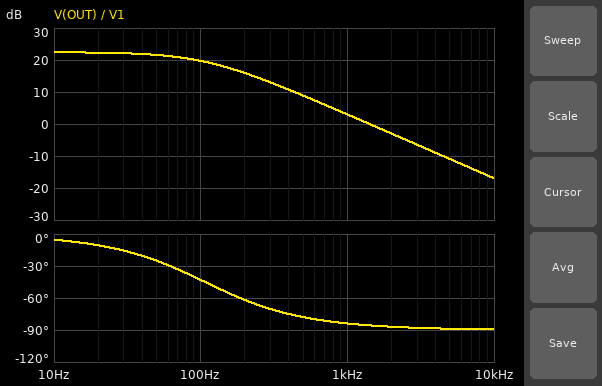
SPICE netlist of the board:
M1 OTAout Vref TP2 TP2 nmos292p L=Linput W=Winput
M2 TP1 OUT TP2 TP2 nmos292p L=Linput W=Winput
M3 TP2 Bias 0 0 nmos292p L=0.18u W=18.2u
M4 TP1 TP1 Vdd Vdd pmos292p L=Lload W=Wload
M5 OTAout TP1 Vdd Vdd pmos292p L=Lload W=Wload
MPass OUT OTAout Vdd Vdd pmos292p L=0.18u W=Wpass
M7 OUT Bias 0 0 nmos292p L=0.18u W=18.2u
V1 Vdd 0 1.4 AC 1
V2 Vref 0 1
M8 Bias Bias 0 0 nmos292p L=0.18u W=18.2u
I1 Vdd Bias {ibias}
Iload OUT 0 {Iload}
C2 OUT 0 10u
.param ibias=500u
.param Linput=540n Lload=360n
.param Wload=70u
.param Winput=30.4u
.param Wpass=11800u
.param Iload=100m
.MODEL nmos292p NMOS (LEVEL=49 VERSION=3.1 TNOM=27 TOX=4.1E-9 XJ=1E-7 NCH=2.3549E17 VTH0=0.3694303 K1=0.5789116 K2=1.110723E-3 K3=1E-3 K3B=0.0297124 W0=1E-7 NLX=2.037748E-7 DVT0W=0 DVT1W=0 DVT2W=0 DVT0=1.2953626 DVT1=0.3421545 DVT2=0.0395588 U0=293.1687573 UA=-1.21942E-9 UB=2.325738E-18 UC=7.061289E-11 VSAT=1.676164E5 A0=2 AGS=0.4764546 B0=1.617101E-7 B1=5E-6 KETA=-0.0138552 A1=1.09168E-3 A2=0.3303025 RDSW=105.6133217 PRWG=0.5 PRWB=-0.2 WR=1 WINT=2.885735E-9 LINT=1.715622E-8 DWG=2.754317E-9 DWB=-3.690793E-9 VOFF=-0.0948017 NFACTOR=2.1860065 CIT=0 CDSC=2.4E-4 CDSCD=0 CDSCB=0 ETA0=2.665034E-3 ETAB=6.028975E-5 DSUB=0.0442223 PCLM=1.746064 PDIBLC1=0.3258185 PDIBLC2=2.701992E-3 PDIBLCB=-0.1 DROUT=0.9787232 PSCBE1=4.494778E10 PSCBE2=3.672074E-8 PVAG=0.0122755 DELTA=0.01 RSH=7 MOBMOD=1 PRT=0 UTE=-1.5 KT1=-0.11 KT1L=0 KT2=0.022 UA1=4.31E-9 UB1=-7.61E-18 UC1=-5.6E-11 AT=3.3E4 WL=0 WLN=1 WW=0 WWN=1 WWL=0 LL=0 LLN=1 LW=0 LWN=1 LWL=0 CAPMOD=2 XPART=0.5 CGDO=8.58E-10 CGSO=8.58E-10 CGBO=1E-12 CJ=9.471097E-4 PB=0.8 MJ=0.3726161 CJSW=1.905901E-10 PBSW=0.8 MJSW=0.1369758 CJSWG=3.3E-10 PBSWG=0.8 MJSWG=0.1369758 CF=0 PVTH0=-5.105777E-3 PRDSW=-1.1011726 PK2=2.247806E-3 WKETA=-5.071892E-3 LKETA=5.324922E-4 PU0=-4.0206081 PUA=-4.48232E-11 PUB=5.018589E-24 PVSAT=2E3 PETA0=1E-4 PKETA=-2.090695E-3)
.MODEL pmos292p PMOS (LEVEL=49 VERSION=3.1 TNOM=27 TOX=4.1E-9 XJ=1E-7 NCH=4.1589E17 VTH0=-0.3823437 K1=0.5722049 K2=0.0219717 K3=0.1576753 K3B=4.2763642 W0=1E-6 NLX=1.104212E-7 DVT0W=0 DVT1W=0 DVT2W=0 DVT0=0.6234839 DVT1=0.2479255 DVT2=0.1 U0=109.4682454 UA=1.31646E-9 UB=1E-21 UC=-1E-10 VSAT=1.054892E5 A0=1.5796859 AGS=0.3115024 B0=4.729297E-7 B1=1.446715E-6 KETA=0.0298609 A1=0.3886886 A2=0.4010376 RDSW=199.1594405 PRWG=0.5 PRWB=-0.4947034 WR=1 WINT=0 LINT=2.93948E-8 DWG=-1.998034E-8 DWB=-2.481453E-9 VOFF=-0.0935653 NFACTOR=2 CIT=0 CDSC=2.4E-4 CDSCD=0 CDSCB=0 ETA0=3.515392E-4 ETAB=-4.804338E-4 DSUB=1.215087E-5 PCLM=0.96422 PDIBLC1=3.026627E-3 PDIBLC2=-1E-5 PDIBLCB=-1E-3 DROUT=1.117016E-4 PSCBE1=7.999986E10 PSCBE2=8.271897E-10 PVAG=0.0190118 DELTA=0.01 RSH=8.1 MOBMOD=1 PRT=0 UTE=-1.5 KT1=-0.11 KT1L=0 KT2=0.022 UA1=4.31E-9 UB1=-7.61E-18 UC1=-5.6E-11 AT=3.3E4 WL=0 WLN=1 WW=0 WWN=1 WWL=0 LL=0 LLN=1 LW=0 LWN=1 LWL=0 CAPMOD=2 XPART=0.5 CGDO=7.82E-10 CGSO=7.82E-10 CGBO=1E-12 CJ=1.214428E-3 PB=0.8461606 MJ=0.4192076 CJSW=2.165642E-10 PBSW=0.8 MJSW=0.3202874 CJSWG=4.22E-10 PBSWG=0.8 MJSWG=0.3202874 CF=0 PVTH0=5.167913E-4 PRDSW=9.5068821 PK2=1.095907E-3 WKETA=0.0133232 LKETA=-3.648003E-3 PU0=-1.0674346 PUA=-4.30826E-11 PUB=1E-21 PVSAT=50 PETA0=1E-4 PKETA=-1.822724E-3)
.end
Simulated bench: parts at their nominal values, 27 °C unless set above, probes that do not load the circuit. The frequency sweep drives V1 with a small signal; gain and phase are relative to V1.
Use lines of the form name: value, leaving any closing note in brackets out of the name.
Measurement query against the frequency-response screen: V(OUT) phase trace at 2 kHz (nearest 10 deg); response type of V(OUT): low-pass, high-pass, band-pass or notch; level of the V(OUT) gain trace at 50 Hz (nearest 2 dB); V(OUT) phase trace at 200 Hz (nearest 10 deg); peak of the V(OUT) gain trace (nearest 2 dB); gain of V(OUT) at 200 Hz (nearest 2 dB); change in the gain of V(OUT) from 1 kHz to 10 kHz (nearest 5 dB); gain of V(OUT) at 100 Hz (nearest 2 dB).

V(OUT) phase trace at 2 kHz: -90 deg
response type of V(OUT): low-pass, high-pass, band-pass or notch: low-pass
level of the V(OUT) gain trace at 50 Hz: 22 dB
V(OUT) phase trace at 200 Hz: -60 deg
peak of the V(OUT) gain trace: 22 dB
gain of V(OUT) at 200 Hz: 16 dB
change in the gain of V(OUT) from 1 kHz to 10 kHz: -20 dB
gain of V(OUT) at 100 Hz: 20 dB
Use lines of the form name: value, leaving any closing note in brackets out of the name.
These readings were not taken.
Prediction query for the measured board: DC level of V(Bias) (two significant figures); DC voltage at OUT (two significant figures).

DC level of V(Bias): 660 mV
DC voltage at OUT: -3.1 V
